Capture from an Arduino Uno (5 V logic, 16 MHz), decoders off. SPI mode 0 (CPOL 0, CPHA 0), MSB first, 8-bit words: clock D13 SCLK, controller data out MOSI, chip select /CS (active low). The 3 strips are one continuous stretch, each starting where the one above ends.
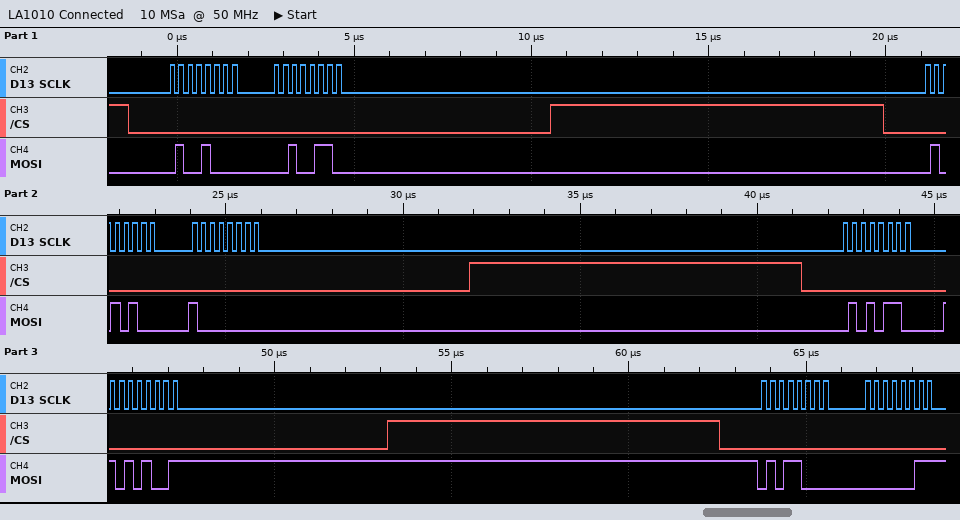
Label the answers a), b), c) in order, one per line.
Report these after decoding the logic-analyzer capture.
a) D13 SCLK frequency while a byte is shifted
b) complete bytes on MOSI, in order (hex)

a) 4 MHz
b) 0x48 0x26 0x54 0x80 0x56 0xA9 0x58 0x03
